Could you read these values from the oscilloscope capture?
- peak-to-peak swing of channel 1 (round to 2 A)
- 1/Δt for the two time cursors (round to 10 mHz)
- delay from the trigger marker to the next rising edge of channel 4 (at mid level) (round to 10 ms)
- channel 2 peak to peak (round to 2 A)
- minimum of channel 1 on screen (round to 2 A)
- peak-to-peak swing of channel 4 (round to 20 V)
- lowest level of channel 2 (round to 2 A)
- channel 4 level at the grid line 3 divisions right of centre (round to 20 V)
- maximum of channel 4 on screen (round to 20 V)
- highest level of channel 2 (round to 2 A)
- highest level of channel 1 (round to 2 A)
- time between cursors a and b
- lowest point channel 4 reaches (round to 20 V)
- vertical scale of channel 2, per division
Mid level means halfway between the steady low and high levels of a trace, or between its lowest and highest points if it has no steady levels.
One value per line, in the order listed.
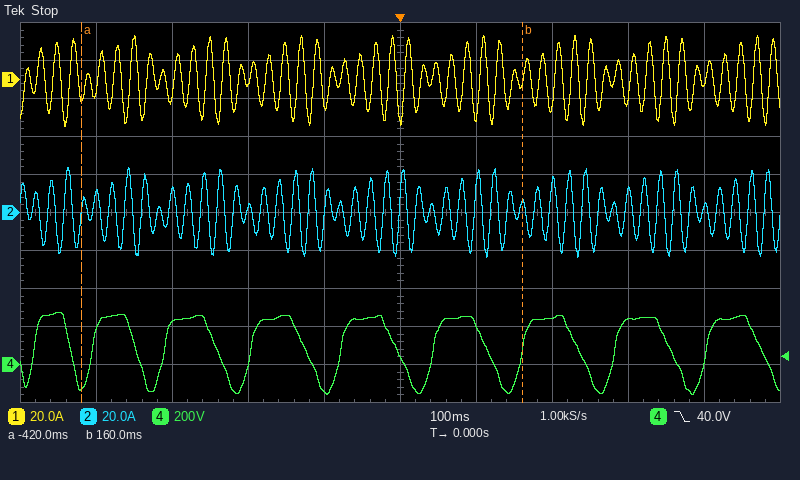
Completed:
48 A
1.72 Hz
40 ms
48 A
-24 A
440 V
-24 A
240 V
280 V
24 A
24 A
580 ms
-160 V
20 A
